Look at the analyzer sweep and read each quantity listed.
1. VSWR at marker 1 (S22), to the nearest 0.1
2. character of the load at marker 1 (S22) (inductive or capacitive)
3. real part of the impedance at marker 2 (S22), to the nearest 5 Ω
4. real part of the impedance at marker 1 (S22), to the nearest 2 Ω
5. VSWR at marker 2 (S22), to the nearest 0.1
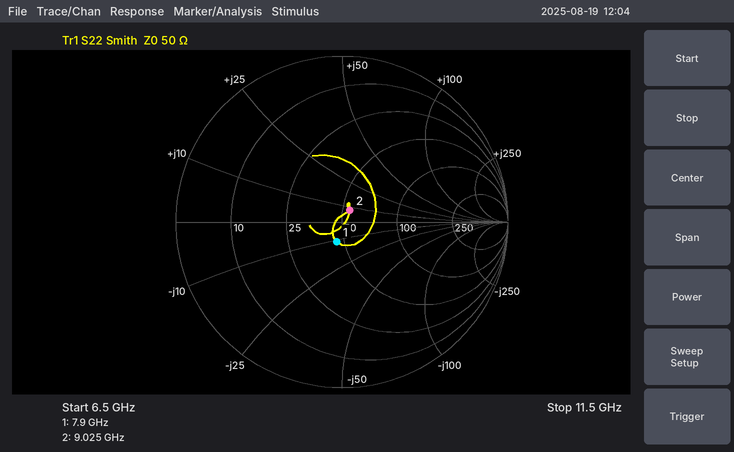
1.3
capacitive
55 Ω
46 Ω
1.2
